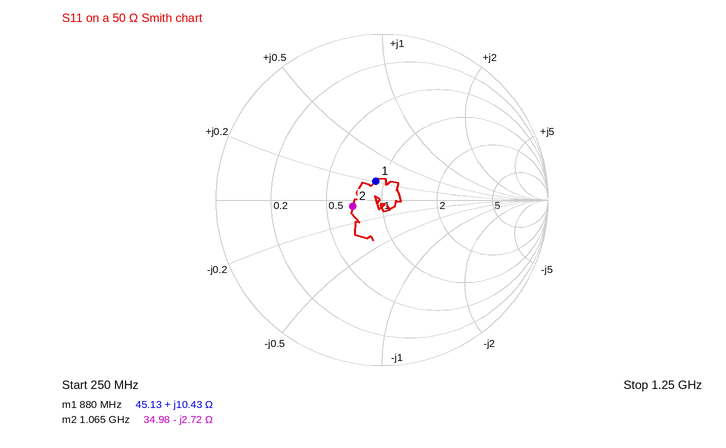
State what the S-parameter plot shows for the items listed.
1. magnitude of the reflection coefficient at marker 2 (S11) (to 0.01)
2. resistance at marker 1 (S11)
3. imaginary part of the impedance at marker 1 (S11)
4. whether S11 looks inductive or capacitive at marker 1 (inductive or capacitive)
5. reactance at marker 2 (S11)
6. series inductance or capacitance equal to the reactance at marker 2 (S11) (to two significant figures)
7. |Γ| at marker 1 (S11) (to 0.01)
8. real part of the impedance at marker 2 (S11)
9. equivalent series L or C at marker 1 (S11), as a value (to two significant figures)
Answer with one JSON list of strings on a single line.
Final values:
["0.18", "45.13 Ω", "+10.43 Ω", "inductive", "-2.72 Ω", "55 pF", "0.12", "34.98 Ω", "1.9 nH"]
